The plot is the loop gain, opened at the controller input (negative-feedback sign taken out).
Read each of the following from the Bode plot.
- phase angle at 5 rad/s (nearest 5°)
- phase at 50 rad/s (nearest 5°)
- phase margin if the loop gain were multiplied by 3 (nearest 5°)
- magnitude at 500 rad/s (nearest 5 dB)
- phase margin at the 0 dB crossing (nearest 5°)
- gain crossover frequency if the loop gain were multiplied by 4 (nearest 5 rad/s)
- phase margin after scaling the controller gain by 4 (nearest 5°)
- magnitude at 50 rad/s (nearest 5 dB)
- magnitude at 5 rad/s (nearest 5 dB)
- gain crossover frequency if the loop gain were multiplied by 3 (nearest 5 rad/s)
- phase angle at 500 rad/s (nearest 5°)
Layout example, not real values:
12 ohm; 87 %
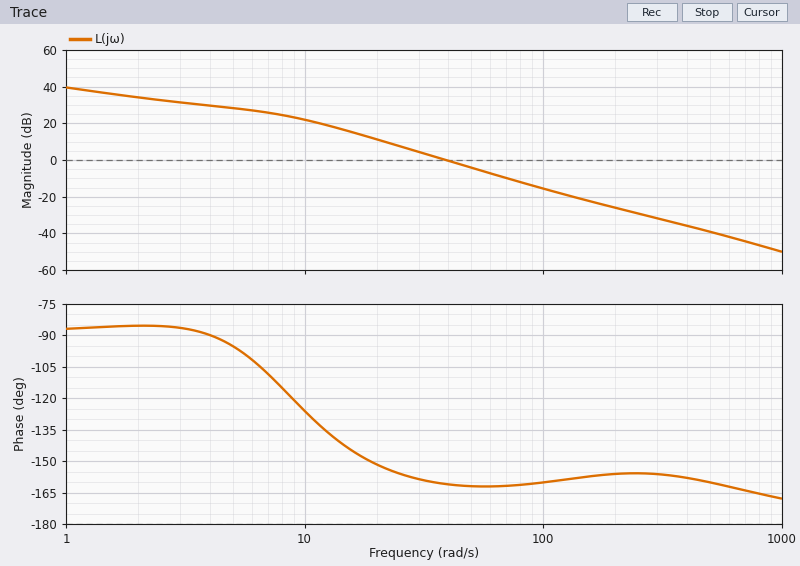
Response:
-95°; -160°; 20°; -40 dB; 20°; 80 rad/s; 20°; -5 dB; 30 dB; 70 rad/s; -160°
